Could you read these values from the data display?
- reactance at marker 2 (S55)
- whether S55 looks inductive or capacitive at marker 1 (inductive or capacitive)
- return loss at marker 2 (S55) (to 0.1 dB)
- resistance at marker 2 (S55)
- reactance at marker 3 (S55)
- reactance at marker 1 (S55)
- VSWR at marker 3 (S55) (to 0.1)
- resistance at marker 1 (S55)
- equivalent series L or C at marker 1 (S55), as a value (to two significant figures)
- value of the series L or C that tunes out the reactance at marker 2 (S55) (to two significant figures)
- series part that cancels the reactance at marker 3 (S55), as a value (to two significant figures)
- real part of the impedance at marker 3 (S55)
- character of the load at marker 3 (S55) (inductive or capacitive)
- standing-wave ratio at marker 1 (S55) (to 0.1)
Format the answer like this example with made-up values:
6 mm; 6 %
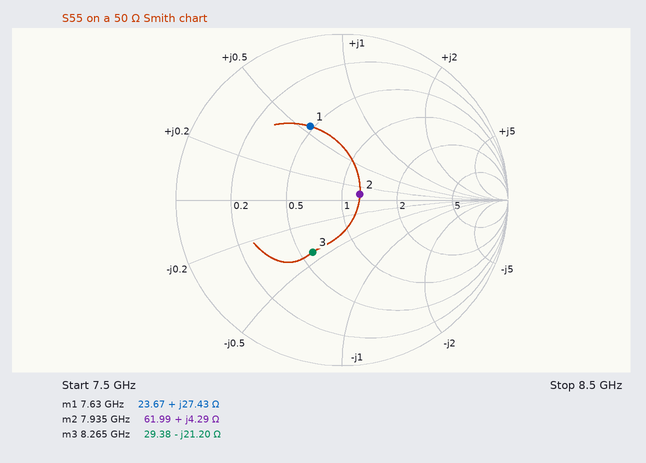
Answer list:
+4.29 Ω; inductive; 18.9 dB; 61.99 Ω; -21.20 Ω; +27.43 Ω; 2.1; 23.67 Ω; 570 pH; 4.7 pF; 410 pH; 29.38 Ω; capacitive; 2.9
